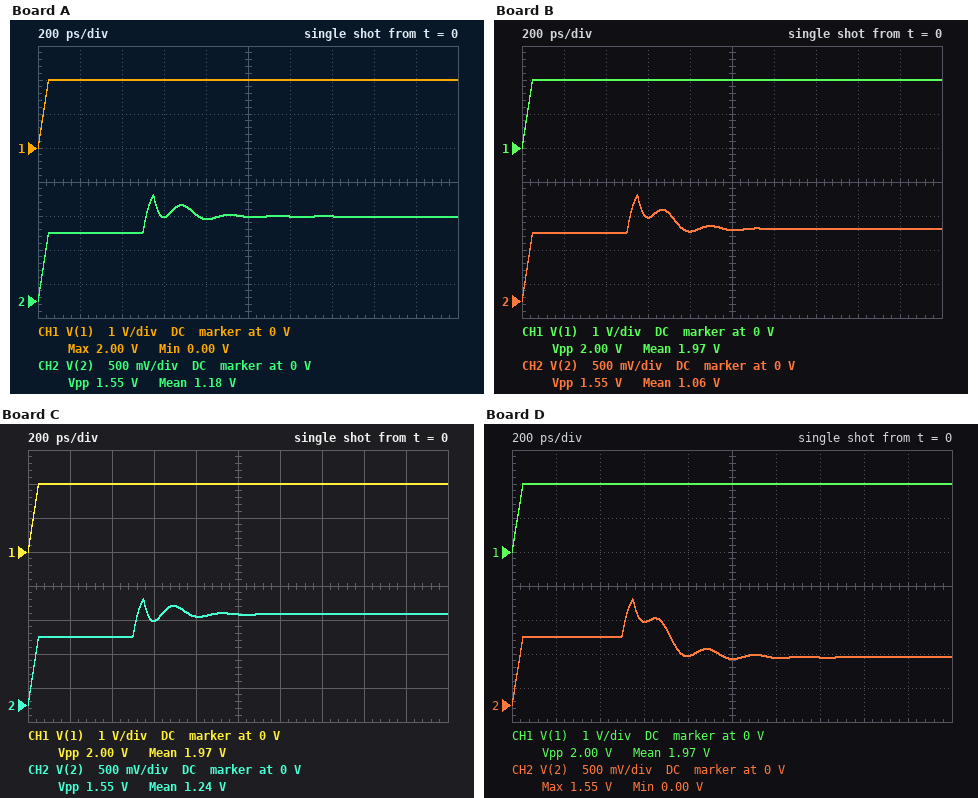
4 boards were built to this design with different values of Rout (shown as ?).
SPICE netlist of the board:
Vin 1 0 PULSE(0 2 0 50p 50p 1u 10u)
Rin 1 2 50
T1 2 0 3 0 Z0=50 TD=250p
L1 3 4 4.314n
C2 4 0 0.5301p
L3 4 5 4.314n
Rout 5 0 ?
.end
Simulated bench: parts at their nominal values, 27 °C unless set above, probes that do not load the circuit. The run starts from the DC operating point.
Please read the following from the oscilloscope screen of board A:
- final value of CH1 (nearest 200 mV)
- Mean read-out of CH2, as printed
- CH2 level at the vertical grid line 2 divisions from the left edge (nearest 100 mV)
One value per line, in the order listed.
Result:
2.0 V
1.18 V
1.0 V
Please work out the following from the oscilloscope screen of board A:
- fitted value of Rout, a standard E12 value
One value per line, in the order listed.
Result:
82 Ω
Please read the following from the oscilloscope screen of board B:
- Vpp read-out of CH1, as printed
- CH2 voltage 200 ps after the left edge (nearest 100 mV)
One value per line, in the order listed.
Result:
2.00 V
1.0 V
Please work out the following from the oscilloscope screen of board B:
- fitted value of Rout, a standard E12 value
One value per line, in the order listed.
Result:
56 Ω
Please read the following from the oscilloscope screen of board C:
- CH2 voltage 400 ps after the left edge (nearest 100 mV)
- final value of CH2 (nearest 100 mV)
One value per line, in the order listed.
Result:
1.0 V
1.3 V
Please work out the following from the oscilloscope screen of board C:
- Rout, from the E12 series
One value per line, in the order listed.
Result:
100 Ω
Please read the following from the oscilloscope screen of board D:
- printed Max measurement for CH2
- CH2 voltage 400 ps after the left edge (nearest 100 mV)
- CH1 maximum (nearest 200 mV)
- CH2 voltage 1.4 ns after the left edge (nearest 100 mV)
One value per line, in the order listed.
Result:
1.55 V
1.0 V
2.0 V
700 mV
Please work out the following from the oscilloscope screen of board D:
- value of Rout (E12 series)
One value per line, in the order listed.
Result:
27 Ω
